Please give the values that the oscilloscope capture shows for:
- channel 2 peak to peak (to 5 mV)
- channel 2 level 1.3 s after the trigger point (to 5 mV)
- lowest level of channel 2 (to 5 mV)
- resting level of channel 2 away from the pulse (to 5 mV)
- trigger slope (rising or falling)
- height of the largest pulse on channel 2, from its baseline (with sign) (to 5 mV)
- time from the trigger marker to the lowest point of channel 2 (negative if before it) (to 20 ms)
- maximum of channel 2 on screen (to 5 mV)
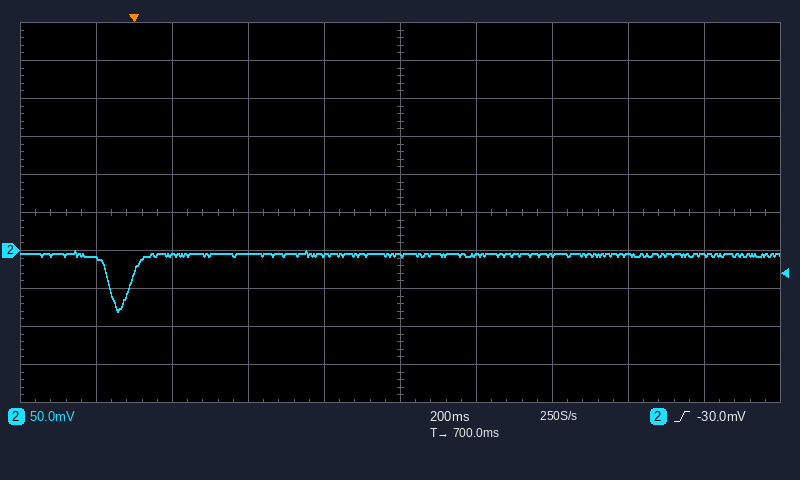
80 mV
-5 mV
-80 mV
-5 mV
rising
-75 mV
-40 ms
0 mV
